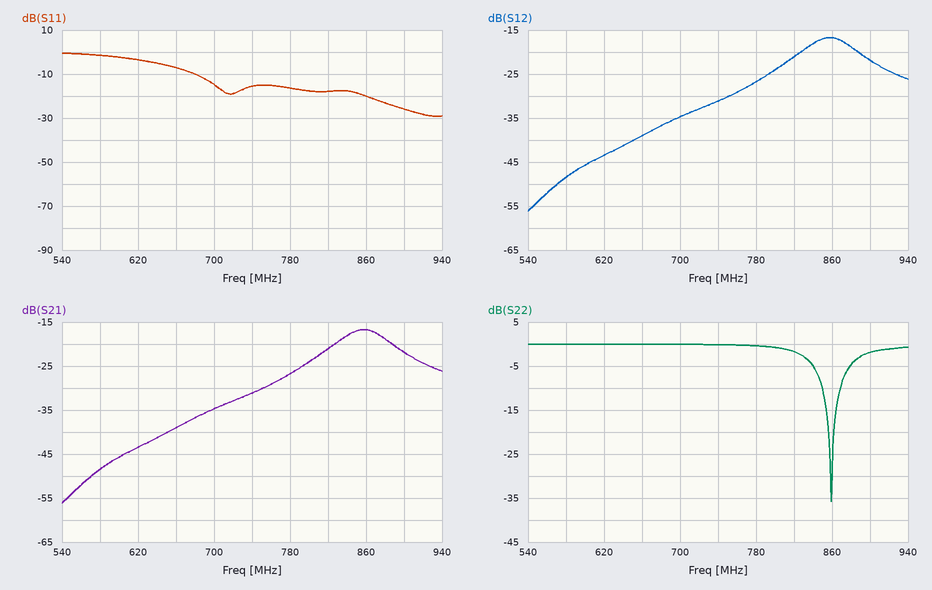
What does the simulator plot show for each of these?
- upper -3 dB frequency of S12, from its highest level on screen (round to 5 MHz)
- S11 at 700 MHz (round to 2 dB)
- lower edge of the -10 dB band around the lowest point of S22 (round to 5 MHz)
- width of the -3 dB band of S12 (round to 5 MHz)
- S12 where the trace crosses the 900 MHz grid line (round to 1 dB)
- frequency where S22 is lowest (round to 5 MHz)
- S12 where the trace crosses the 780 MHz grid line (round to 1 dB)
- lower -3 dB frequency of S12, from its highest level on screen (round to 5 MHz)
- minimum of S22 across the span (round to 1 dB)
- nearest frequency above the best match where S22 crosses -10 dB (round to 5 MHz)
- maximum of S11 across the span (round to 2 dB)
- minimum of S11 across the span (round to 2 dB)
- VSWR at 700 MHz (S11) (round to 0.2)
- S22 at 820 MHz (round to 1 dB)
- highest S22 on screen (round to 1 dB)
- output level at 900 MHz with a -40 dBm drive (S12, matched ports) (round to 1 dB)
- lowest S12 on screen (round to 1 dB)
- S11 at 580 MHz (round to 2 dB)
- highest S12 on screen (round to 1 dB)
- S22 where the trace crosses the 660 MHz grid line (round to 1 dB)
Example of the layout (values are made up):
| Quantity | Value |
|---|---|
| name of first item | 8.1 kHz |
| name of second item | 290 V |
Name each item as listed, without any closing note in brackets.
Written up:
| Quantity | Value |
|---|---|
| upper -3 dB frequency of S12, from its highest level on screen | 885 MHz |
| S11 at 700 MHz | -14 dB |
| lower edge of the -10 dB band around the lowest point of S22 | 850 MHz |
| width of the -3 dB band of S12 | 55 MHz |
| S12 where the trace crosses the 900 MHz grid line | -22 dB |
| frequency where S22 is lowest | 860 MHz |
| S12 where the trace crosses the 780 MHz grid line | -27 dB |
| lower -3 dB frequency of S12, from its highest level on screen | 830 MHz |
| minimum of S22 across the span | -36 dB |
| nearest frequency above the best match where S22 crosses -10 dB | 870 MHz |
| maximum of S11 across the span | 0 dB |
| minimum of S11 across the span | -30 dB |
| VSWR at 700 MHz (S11) | 1.4 |
| S22 at 820 MHz | -2 dB |
| highest S22 on screen | 0 dB |
| output level at 900 MHz with a -40 dBm drive (S12, matched ports) | -62 dBm |
| lowest S12 on screen | -56 dB |
| S11 at 580 MHz | -2 dB |
| highest S12 on screen | -17 dB |
| S22 where the trace crosses the 660 MHz grid line | 0 dB |
